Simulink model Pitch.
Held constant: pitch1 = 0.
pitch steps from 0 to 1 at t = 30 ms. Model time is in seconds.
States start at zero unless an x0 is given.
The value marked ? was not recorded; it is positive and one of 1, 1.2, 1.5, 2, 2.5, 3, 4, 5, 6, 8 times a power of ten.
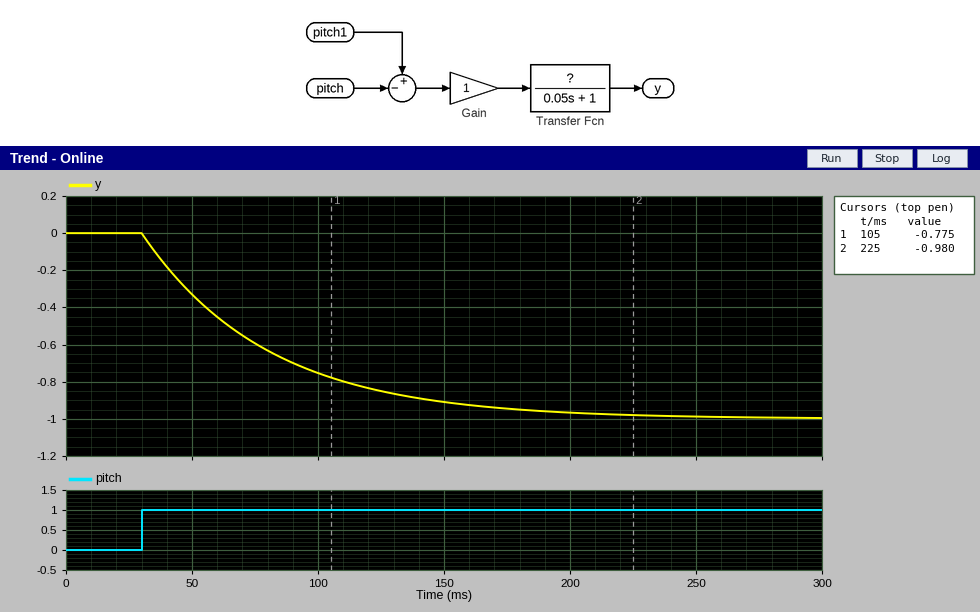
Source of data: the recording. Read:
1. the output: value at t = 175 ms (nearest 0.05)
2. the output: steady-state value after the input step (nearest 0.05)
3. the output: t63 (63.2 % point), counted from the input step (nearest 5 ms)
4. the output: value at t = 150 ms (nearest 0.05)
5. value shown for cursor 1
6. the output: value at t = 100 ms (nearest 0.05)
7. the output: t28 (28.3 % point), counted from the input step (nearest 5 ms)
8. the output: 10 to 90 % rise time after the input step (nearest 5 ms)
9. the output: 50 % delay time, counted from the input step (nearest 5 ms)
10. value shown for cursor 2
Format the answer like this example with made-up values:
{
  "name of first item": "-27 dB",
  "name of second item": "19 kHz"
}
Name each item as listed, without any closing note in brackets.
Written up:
{
  "the output: value at t = 175 ms": "-0.95",
  "the output: steady-state value after the input step": "-1.00",
  "the output: t63 (63.2 % point), counted from the input step": "50 ms",
  "the output: value at t = 150 ms": "-0.90",
  "value shown for cursor 1": "-0.775",
  "the output: value at t = 100 ms": "-0.75",
  "the output: t28 (28.3 % point), counted from the input step": "15 ms",
  "the output: 10 to 90 % rise time after the input step": "110 ms",
  "the output: 50 % delay time, counted from the input step": "35 ms",
  "value shown for cursor 2": "-0.980"
}
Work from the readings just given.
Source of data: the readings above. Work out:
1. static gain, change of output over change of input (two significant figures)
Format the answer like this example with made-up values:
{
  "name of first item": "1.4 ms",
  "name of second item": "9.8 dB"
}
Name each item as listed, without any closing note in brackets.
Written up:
{
  "static gain, change of output over change of input": "-1.0"
}
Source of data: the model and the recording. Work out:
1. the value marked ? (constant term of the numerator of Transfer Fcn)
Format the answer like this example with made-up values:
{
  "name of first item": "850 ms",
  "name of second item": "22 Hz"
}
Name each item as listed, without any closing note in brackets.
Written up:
{
  "the value marked ?": "1"
}
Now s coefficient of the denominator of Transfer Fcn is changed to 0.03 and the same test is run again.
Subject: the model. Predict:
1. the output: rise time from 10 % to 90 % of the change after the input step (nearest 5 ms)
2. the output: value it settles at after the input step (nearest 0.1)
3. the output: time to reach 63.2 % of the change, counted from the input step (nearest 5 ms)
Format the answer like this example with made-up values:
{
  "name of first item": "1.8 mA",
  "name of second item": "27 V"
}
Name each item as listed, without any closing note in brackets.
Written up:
{
  "the output: rise time from 10 % to 90 % of the change after the input step": "65 ms",
  "the output: value it settles at after the input step": "-1.0",
  "the output: time to reach 63.2 % of the change, counted from the input step": "30 ms"
}
